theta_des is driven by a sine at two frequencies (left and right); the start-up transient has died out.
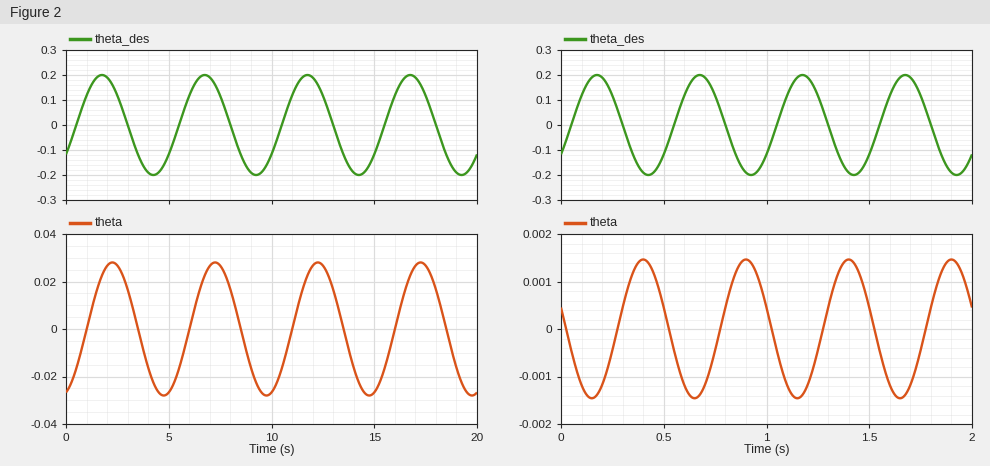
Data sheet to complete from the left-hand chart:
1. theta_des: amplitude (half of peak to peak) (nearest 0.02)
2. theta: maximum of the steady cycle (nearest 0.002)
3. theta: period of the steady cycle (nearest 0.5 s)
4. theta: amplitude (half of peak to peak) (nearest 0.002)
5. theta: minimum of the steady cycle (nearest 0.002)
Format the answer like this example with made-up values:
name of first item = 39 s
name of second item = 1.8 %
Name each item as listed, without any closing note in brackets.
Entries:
theta_des: amplitude (half of peak to peak) = 0.20
theta: maximum of the steady cycle = 0.028
theta: period of the steady cycle = 5.0 s
theta: amplitude (half of peak to peak) = 0.028
theta: minimum of the steady cycle = -0.028
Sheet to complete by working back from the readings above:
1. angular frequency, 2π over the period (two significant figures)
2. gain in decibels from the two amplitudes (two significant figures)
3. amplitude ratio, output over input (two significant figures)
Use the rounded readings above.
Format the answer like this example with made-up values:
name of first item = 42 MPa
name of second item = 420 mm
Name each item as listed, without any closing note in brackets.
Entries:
angular frequency, 2π over the period = 1.3 rad/s
gain in decibels from the two amplitudes = -17 dB
amplitude ratio, output over input = 0.14
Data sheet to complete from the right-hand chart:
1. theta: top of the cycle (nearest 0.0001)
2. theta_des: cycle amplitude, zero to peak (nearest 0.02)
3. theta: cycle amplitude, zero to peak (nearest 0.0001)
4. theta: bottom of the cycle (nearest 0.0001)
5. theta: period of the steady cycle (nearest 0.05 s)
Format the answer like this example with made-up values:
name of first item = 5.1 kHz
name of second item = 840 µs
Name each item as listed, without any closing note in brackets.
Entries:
theta: top of the cycle = 0.0015
theta_des: cycle amplitude, zero to peak = 0.20
theta: cycle amplitude, zero to peak = 0.0015
theta: bottom of the cycle = -0.0015
theta: period of the steady cycle = 0.50 s
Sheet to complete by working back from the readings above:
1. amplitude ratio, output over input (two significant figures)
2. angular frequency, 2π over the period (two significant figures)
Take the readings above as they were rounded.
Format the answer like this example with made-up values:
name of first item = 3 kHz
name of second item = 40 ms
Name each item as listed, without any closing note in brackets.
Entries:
amplitude ratio, output over input = 0.0075
angular frequency, 2π over the period = 13 rad/s
